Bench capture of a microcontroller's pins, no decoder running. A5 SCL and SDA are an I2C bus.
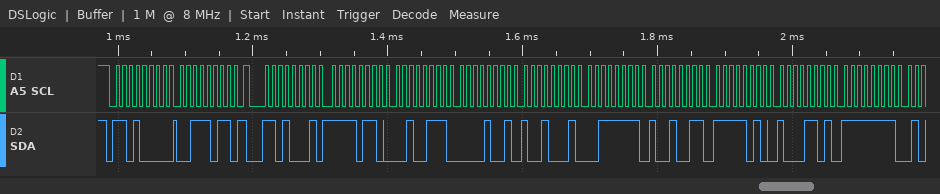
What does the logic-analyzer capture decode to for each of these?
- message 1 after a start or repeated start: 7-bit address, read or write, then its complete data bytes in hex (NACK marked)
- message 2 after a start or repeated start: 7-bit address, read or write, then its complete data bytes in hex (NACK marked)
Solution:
0x68 write: 3B
0x68 read: F6 27 09 91 3F 93 FA 8D FF
